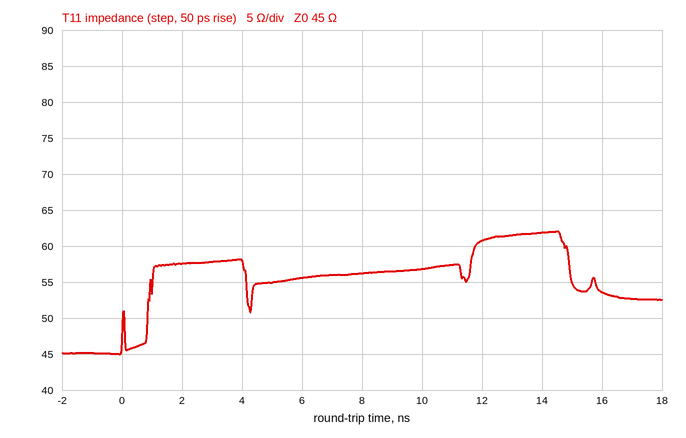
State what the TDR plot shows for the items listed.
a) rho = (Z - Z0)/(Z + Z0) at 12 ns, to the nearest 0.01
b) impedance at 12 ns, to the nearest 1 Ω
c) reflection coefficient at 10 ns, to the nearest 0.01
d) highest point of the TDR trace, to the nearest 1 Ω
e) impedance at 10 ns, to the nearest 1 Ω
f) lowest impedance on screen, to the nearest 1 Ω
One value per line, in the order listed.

+0.15
61 Ω
+0.12
62 Ω
57 Ω
45 Ω
